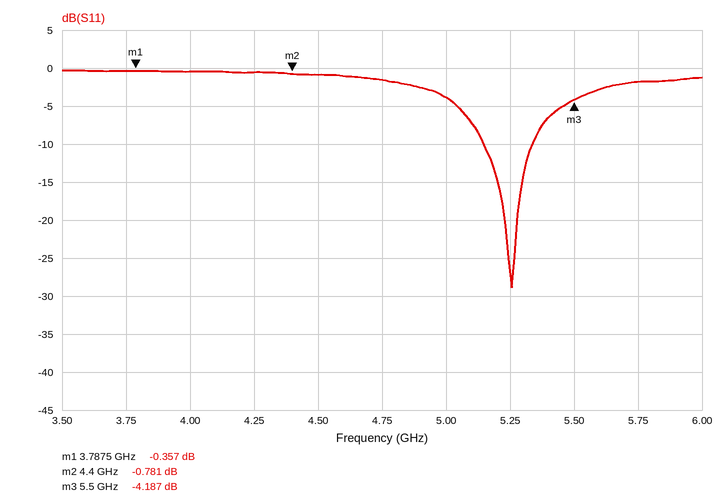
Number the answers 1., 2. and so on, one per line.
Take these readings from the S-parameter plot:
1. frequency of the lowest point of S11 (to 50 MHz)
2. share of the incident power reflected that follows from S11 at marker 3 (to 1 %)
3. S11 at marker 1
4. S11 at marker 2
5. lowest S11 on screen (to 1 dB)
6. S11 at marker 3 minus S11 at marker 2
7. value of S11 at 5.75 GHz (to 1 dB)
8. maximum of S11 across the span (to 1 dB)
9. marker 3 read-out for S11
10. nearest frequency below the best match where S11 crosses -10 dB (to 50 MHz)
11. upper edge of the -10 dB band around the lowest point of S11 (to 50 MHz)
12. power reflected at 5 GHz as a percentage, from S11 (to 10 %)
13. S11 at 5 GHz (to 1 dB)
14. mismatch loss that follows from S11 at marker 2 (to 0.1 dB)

1. 5.25 GHz
2. 38 %
3. -0.357 dB
4. -0.781 dB
5. -29 dB
6. -3.406 dB
7. -2 dB
8. 0 dB
9. -4.187 dB
10. 5.15 GHz
11. 5.35 GHz
12. 40 %
13. -4 dB
14. 7.8 dB
